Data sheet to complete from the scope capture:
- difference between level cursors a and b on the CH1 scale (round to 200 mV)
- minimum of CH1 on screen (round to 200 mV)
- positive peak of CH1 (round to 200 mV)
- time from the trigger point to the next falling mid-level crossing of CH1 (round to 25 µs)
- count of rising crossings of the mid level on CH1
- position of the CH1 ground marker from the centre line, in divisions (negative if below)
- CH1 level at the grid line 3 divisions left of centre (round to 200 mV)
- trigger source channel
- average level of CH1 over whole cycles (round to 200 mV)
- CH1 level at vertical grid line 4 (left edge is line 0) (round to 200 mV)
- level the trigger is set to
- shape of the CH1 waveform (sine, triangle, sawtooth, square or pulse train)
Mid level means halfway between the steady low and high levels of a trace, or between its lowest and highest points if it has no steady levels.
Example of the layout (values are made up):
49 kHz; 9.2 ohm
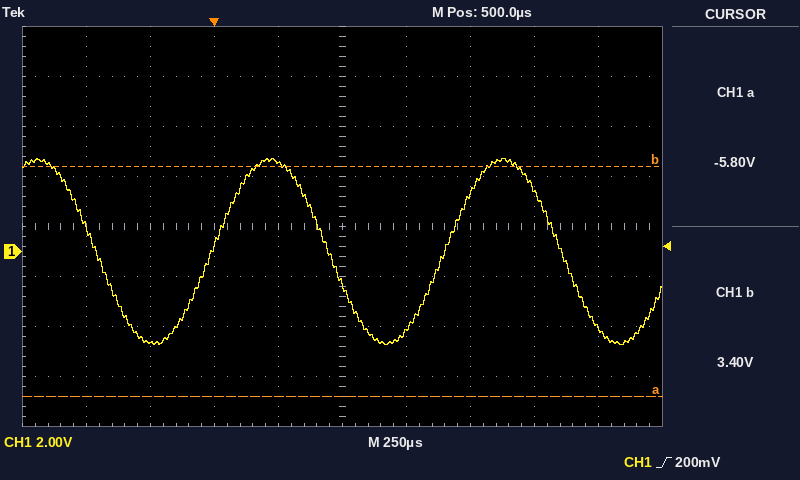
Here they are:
9.2 V; -3.8 V; 3.8 V; 450 µs; 2; -0.5 div; -3.6 V; CH1; 0.0 V; 3.6 V; 200 mV; sine
